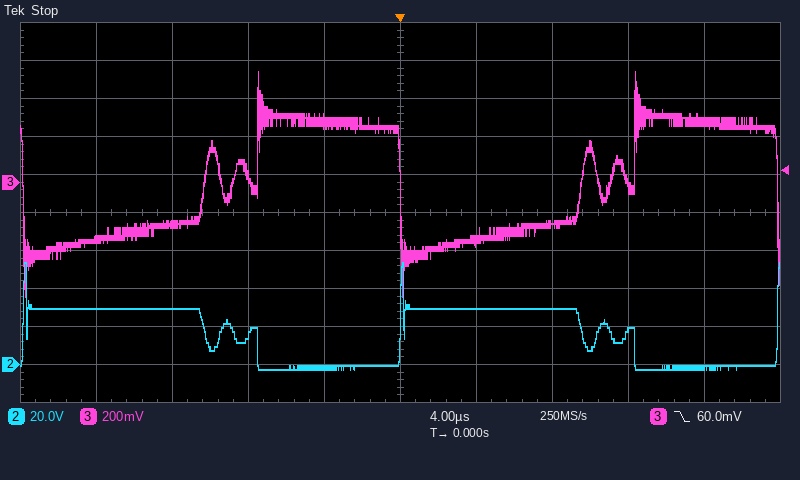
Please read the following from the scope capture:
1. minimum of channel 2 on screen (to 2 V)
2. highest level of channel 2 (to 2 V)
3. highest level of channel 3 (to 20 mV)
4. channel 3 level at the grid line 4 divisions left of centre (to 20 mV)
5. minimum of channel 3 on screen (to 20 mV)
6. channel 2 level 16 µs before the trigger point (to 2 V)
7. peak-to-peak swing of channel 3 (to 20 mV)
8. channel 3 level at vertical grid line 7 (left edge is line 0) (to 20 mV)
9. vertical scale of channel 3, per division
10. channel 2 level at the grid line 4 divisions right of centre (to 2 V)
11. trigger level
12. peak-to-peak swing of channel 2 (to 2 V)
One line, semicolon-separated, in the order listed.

-2 V; 54 V; 580 mV; -300 mV; -600 mV; 30 V; 1.18 V; -220 mV; 200 mV; -2 V; 60.0 mV; 56 V
